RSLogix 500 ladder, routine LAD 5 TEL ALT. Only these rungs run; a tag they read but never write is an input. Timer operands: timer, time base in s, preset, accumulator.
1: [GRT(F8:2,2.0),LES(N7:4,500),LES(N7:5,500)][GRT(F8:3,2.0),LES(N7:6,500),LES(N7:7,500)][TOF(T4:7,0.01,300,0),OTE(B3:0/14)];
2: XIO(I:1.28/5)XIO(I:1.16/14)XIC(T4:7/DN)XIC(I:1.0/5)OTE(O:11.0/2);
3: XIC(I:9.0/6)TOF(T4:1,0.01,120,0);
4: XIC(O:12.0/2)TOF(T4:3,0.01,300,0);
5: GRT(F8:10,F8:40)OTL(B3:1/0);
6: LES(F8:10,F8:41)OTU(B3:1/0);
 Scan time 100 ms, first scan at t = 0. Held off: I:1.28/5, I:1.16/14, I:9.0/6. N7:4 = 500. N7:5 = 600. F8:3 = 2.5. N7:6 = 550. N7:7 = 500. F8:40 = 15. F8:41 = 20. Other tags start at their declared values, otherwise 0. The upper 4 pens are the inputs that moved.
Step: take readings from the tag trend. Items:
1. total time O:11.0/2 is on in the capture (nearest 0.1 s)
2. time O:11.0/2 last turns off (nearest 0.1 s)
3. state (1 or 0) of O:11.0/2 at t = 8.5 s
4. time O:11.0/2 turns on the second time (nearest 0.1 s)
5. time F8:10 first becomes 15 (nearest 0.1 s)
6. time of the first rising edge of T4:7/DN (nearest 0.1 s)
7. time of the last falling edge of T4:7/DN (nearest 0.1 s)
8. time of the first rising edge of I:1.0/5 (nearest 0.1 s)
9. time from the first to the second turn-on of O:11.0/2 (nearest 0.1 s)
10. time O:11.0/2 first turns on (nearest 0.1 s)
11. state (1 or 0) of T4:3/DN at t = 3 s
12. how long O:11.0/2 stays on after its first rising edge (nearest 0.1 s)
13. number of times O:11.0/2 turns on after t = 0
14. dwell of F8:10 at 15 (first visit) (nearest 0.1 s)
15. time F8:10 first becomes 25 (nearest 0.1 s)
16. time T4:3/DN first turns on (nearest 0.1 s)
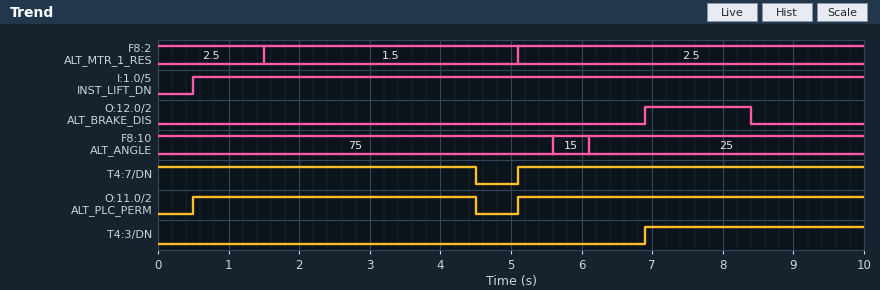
8.9 s
4.5 s
1
5.1 s
5.6 s
5.1 s
4.5 s
0.5 s
4.6 s
0.5 s
0
4.0 s
2
0.5 s
6.1 s
6.9 s
